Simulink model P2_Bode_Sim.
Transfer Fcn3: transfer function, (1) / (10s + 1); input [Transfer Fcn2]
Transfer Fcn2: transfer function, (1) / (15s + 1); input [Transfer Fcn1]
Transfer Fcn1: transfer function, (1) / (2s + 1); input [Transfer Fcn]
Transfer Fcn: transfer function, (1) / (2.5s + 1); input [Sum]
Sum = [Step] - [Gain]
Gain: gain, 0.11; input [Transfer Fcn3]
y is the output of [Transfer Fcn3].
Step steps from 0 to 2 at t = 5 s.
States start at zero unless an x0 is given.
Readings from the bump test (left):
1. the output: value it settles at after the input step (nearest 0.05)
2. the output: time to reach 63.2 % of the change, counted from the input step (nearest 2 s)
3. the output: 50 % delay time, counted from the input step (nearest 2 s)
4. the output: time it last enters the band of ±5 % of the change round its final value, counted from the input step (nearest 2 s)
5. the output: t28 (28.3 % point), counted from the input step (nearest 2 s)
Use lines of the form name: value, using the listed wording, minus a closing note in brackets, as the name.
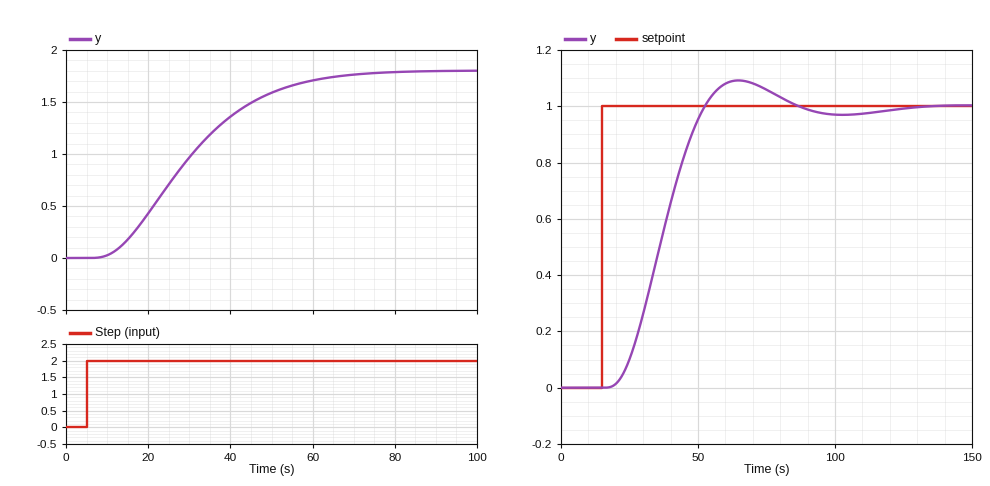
the output: value it settles at after the input step: 1.80
the output: time to reach 63.2 % of the change, counted from the input step: 28 s
the output: 50 % delay time, counted from the input step: 24 s
the output: time it last enters the band of ±5 % of the change round its final value, counted from the input step: 56 s
the output: t28 (28.3 % point), counted from the input step: 16 s
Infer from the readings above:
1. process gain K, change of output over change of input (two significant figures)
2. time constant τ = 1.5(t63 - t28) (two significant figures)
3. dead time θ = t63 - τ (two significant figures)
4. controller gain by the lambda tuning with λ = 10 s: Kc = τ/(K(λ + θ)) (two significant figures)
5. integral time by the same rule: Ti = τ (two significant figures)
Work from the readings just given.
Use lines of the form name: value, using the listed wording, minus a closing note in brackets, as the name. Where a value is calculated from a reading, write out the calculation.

process gain K, change of output over change of input: (1.8 - 0) / 2 = 0.90
time constant τ = 1.5(t63 - t28): 1.5 × (28 - 16) = 18 s
dead time θ = t63 - τ: 28 - 18 = 10 s
controller gain by the lambda tuning with λ = 10 s: Kc = τ/(K(λ + θ)): 18 / (0.9 × (10 + 10)) = 1.0
integral time by the same rule: Ti = τ: 18 s
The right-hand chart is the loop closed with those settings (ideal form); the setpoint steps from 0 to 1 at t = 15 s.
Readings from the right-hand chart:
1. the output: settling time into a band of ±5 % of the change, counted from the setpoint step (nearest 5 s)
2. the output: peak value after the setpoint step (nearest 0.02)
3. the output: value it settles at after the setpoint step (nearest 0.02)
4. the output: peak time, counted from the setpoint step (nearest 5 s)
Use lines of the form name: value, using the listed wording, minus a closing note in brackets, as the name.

the output: settling time into a band of ±5 % of the change, counted from the setpoint step: 60 s
the output: peak value after the setpoint step: 1.10
the output: value it settles at after the setpoint step: 1.00
the output: peak time, counted from the setpoint step: 50 s
